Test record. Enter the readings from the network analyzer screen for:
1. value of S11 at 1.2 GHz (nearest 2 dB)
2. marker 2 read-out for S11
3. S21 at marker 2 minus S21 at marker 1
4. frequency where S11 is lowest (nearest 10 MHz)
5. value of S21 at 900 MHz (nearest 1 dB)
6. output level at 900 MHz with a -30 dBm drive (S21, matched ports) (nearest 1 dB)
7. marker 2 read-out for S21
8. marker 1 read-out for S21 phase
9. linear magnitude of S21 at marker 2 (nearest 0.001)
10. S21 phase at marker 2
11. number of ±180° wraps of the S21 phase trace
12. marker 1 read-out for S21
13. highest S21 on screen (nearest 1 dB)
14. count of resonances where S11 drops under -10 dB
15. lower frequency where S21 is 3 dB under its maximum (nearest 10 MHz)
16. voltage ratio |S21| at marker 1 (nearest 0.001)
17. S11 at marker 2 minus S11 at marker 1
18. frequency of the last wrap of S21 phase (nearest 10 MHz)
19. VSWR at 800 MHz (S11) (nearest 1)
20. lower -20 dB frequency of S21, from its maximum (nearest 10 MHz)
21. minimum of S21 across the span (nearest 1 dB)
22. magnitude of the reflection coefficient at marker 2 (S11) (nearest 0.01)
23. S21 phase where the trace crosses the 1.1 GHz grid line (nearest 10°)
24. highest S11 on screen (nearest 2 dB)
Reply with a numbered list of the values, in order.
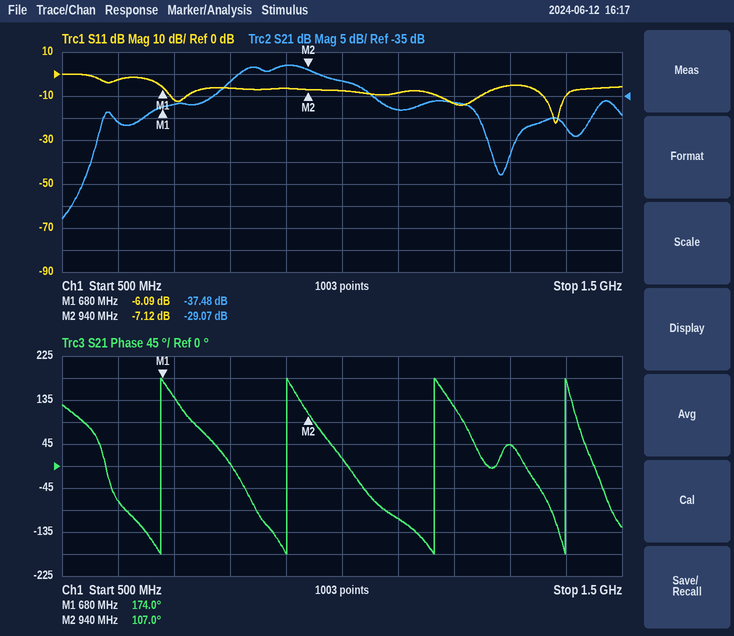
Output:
1. -14 dB
2. -7.12 dB
3. 8.41 dB
4. 1.38 GHz
5. -28 dB
6. -58 dBm
7. -29.07 dB
8. 174.0°
9. 0.035
10. 107.0°
11. 4
12. -37.48 dB
13. -28 dB
14. 3
15. 810 MHz
16. 0.013
17. -1.03 dB
18. 1.40 GHz
19. 3
20. 560 MHz
21. -63 dB
22. 0.44
23. -110°
24. 0 dB
